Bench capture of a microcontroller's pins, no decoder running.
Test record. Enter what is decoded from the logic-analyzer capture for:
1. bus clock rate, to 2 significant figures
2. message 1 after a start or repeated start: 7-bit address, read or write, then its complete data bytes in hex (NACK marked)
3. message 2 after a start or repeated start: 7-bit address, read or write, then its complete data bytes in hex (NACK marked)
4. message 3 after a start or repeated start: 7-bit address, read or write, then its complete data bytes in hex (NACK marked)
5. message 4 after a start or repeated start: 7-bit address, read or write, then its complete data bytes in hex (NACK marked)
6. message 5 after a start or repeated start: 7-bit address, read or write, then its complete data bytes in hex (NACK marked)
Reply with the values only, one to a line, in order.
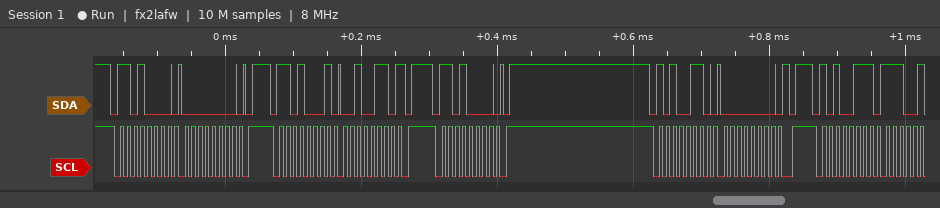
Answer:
100 kHz
0x68 write: 00
0x68 read: 26 NACK
0x68 write
0x53 write: 00
0x53 read
